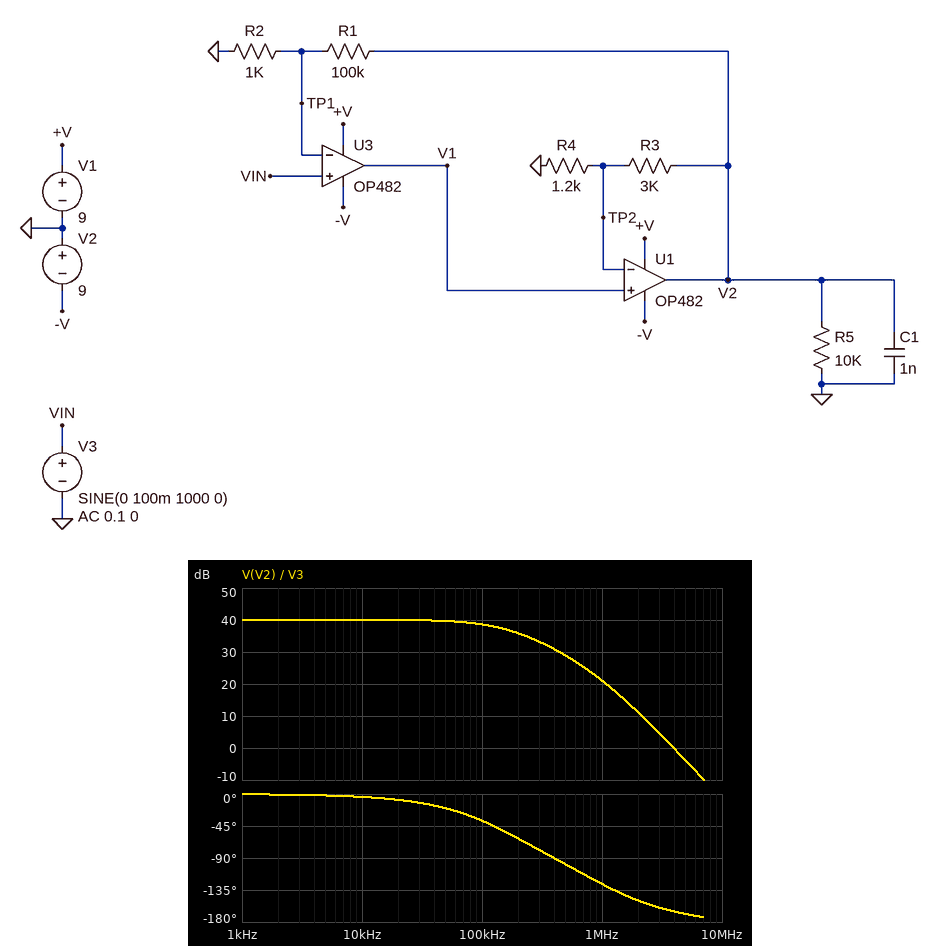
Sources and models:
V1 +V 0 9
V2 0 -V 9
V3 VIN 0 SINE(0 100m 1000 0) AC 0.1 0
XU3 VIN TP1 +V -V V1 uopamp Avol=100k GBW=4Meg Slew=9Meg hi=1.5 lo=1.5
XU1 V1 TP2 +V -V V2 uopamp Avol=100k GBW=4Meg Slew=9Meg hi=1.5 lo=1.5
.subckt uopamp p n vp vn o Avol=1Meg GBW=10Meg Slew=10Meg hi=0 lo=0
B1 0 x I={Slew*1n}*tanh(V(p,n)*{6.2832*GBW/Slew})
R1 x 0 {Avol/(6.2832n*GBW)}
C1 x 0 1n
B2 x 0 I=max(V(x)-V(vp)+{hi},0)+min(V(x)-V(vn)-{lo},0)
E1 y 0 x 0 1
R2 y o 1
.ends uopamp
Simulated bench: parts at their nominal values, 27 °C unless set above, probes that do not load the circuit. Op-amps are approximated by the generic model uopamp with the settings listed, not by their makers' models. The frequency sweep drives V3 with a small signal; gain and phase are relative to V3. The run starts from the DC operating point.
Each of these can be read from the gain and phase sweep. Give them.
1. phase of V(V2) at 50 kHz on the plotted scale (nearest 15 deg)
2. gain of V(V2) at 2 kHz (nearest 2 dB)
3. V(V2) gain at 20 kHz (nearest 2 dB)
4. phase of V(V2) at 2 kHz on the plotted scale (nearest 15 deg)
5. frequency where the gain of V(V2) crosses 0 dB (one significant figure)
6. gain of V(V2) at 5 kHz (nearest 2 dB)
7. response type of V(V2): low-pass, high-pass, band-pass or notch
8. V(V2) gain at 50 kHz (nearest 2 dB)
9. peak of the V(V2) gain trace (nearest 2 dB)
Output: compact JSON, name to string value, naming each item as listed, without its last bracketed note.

{"phase of V(V2) at 50 kHz on the plotted scale": "-15 deg", "gain of V(V2) at 2 kHz": "40 dB", "V(V2) gain at 20 kHz": "40 dB", "phase of V(V2) at 2 kHz on the plotted scale": "0 deg", "frequency where the gain of V(V2) crosses 0 dB": "4 MHz", "gain of V(V2) at 5 kHz": "40 dB", "response type of V(V2): low-pass, high-pass, band-pass or notch": "low-pass", "V(V2) gain at 50 kHz": "40 dB", "peak of the V(V2) gain trace": "40 dB"}
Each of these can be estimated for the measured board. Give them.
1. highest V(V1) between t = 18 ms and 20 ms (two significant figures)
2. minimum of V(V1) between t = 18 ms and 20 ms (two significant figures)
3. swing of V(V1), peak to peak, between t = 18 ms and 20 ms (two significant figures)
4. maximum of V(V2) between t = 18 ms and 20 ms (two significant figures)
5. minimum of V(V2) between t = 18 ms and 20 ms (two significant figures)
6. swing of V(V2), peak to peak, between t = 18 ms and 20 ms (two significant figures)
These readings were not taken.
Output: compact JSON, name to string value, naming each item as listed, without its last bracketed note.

{"highest V(V1) between t = 18 ms and 20 ms": "7.5 V", "minimum of V(V1) between t = 18 ms and 20 ms": "-7.5 V", "swing of V(V1), peak to peak, between t = 18 ms and 20 ms": "15 V", "maximum of V(V2) between t = 18 ms and 20 ms": "7.5 V", "minimum of V(V2) between t = 18 ms and 20 ms": "-7.5 V", "swing of V(V2), peak to peak, between t = 18 ms and 20 ms": "15 V"}
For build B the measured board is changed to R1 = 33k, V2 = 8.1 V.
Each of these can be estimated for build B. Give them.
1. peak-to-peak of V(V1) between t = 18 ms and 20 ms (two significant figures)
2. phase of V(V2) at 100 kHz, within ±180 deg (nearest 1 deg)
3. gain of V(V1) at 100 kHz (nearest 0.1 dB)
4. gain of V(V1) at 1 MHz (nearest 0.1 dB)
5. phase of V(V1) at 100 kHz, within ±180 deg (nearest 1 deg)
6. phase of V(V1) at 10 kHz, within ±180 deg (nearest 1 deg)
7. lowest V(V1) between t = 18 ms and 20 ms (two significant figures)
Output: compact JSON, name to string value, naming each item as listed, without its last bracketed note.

{"peak-to-peak of V(V1) between t = 18 ms and 20 ms": "1.9 V", "phase of V(V2) at 100 kHz, within ±180 deg": "-14 deg", "gain of V(V1) at 100 kHz": "19.7 dB", "gain of V(V1) at 1 MHz": "13.7 dB", "phase of V(V1) at 100 kHz, within ±180 deg": "-9 deg", "phase of V(V1) at 10 kHz, within ±180 deg": "-1 deg", "lowest V(V1) between t = 18 ms and 20 ms": "-970 mV"}
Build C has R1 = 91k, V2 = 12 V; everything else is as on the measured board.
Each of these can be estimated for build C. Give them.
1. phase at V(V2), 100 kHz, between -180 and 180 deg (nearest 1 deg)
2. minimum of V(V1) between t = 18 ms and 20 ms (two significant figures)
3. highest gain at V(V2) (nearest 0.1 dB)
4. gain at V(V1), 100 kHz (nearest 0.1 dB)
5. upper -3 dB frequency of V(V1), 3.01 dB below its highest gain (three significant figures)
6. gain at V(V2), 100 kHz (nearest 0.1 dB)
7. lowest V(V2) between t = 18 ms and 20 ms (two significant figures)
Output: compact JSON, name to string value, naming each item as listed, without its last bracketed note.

{"phase at V(V2), 100 kHz, between -180 and 180 deg": "-35 deg", "minimum of V(V1) between t = 18 ms and 20 ms": "-2.6 V", "highest gain at V(V2)": "39.3 dB", "gain at V(V1), 100 kHz": "27.2 dB", "upper -3 dB frequency of V(V1), 3.01 dB below its highest gain": "179 kHz", "gain at V(V2), 100 kHz": "38.1 dB", "lowest V(V2) between t = 18 ms and 20 ms": "-9.2 V"}
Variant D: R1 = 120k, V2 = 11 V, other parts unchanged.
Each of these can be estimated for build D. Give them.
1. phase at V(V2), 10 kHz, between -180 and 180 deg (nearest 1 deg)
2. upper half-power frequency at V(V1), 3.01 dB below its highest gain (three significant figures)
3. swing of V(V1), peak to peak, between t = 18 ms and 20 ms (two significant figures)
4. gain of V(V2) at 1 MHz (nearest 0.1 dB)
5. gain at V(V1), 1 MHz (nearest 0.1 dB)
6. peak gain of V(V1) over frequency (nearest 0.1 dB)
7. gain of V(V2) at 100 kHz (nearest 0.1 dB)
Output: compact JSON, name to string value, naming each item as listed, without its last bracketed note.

{"phase at V(V2), 10 kHz, between -180 and 180 deg": "-5 deg", "upper half-power frequency at V(V1), 3.01 dB below its highest gain": "130 kHz", "swing of V(V1), peak to peak, between t = 18 ms and 20 ms": "17 V", "gain of V(V2) at 1 MHz": "21.0 dB", "gain at V(V1), 1 MHz": "12.5 dB", "peak gain of V(V1) over frequency": "30.8 dB", "gain of V(V2) at 100 kHz": "39.6 dB"}
